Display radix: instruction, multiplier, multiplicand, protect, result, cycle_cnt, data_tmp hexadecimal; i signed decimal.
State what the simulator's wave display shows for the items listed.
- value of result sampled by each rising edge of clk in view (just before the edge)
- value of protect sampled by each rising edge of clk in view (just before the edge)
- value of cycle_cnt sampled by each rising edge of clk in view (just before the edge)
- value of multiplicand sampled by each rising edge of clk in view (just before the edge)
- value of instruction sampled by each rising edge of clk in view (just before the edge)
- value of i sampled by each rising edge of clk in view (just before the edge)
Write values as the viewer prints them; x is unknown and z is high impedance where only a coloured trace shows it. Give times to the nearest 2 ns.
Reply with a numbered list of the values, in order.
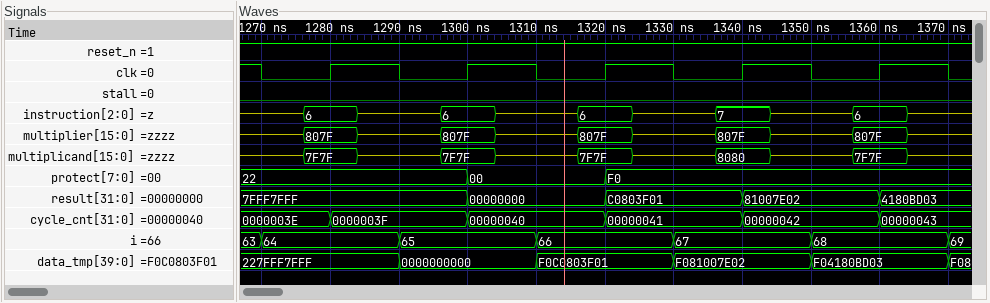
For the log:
1. 7FFF7FFF, 7FFF7FFF, 00000000, C0803F01, 81007E02
2. 22, 22, 00, F0, F0
3. 0000003E, 0000003F, 00000040, 00000041, 00000042
4. 7F7F, 7F7F, 7F7F, 8080, 7F7F
5. 6, 6, 6, 7, 6
6. 64, 65, 66, 67, 68
